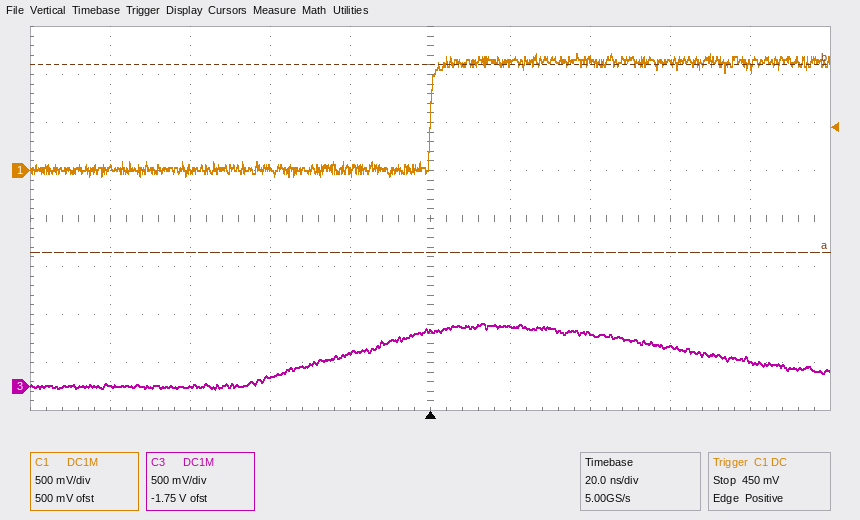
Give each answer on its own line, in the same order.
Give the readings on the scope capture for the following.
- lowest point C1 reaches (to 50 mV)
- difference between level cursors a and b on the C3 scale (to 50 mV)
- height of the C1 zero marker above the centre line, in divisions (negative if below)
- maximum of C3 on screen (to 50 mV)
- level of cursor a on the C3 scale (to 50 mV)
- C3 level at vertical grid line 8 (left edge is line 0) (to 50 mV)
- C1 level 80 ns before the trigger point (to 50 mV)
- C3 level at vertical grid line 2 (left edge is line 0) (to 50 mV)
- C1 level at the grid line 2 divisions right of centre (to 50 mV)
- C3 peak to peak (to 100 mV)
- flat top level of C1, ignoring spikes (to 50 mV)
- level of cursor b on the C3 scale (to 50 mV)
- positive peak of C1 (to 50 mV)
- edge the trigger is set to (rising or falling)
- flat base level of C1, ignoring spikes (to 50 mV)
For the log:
-50 mV
1.95 V
+1.0 div
650 mV
1.40 V
400 mV
0 mV
0 mV
1.15 V
700 mV
1.15 V
3.35 V
1.20 V
rising
0 mV
